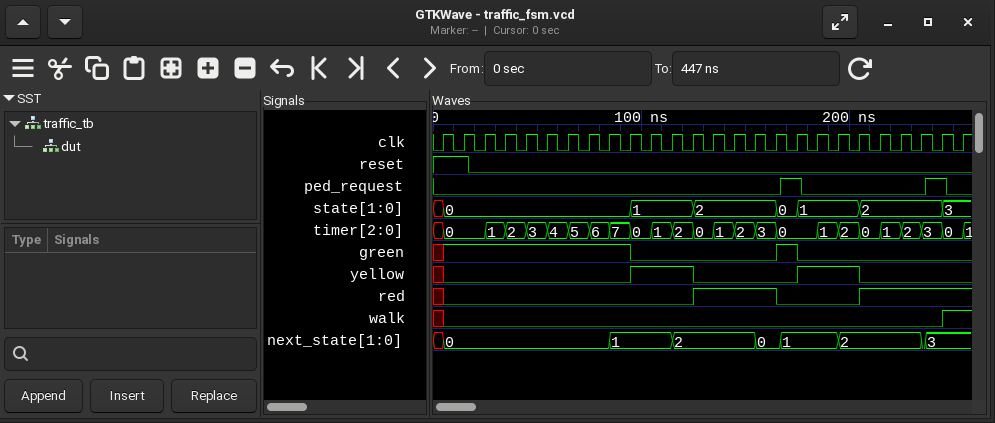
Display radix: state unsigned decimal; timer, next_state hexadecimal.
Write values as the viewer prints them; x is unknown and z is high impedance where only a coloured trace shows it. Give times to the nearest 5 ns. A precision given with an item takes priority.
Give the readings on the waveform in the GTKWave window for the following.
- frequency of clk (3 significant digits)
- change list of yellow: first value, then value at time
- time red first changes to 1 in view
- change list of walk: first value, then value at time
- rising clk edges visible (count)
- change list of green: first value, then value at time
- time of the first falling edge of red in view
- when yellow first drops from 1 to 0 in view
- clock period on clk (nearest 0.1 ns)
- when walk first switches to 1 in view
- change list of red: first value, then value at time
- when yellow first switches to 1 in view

100 MHz
x, 0 at 5 ns, 1 at 95 ns, 0 at 125 ns, 1 at 175 ns, 0 at 205 ns
125 ns
x, 0 at 5 ns, 1 at 245 ns
26
x, 1 at 5 ns, 0 at 95 ns, 1 at 165 ns, 0 at 175 ns
165 ns
125 ns
10 ns
245 ns
x, 0 at 5 ns, 1 at 125 ns, 0 at 165 ns, 1 at 205 ns
95 ns
